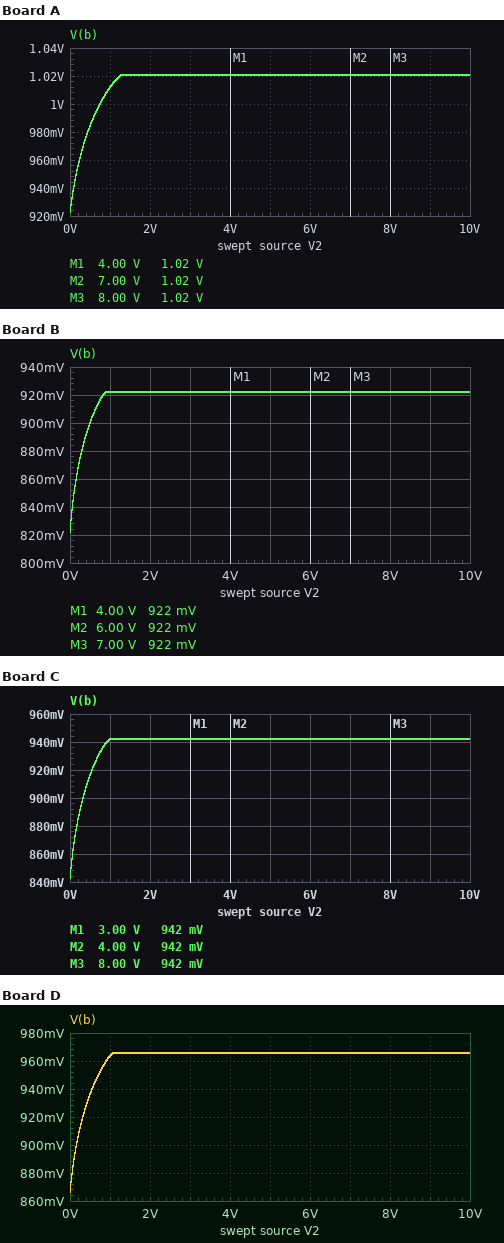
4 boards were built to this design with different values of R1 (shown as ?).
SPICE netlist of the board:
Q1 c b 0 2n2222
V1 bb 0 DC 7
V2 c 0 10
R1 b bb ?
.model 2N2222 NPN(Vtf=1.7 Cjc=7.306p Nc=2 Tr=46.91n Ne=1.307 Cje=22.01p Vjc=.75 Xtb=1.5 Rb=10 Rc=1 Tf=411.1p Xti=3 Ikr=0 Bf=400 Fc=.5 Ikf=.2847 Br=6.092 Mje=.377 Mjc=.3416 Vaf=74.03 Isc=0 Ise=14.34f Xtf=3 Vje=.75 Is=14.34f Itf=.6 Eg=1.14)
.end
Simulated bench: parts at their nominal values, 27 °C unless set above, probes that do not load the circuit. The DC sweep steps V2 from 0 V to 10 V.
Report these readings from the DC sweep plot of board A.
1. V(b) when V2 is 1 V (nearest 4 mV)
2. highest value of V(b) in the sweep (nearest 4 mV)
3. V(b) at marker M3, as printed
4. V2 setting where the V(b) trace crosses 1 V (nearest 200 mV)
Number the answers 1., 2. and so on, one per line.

1. 1.012 V
2. 1.020 V
3. 1.02 V
4. 800 mV
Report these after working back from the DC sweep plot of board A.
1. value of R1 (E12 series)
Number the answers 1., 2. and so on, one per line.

1. 390 Ω
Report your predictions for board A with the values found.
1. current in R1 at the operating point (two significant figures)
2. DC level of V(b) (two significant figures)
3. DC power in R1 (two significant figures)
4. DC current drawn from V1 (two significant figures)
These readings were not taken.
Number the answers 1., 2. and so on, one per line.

1. 15 mA
2. 1.0 V
3. 92 mW
4. 15 mA
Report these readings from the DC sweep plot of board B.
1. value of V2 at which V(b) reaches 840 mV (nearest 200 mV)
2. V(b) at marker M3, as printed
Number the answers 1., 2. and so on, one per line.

1. 0 V
2. 922 mV
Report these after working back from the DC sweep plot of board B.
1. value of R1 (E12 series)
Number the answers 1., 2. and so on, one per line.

1. 820 Ω
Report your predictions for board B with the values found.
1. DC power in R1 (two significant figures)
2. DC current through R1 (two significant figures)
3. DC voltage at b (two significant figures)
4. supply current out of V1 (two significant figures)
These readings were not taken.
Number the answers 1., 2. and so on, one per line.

1. 45 mW
2. 7.4 mA
3. 920 mV
4. 7.4 mA
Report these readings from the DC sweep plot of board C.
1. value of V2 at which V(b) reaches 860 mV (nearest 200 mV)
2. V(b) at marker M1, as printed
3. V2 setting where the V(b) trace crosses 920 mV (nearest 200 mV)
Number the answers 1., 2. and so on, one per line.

1. 0 V
2. 942 mV
3. 600 mV
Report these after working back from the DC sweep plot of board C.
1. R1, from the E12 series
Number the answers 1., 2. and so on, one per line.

1. 680 Ω
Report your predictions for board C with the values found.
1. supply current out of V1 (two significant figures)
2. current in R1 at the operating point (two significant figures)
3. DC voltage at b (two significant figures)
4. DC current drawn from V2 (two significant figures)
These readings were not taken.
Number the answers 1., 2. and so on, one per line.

1. 8.9 mA
2. 8.9 mA
3. 940 mV
4. 890 mA
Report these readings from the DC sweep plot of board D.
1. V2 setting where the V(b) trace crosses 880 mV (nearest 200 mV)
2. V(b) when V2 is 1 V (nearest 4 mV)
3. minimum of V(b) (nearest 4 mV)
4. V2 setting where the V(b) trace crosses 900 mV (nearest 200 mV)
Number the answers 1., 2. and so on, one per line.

1. 0 V
2. 964 mV
3. 868 mV
4. 200 mV
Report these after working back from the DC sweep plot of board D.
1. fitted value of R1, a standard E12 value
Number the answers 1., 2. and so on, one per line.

1. 560 Ω
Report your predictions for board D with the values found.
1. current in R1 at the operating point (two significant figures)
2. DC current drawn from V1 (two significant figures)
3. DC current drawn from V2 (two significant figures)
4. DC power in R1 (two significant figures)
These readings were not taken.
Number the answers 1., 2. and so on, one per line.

1. 11 mA
2. 11 mA
3. 990 mA
4. 65 mW
